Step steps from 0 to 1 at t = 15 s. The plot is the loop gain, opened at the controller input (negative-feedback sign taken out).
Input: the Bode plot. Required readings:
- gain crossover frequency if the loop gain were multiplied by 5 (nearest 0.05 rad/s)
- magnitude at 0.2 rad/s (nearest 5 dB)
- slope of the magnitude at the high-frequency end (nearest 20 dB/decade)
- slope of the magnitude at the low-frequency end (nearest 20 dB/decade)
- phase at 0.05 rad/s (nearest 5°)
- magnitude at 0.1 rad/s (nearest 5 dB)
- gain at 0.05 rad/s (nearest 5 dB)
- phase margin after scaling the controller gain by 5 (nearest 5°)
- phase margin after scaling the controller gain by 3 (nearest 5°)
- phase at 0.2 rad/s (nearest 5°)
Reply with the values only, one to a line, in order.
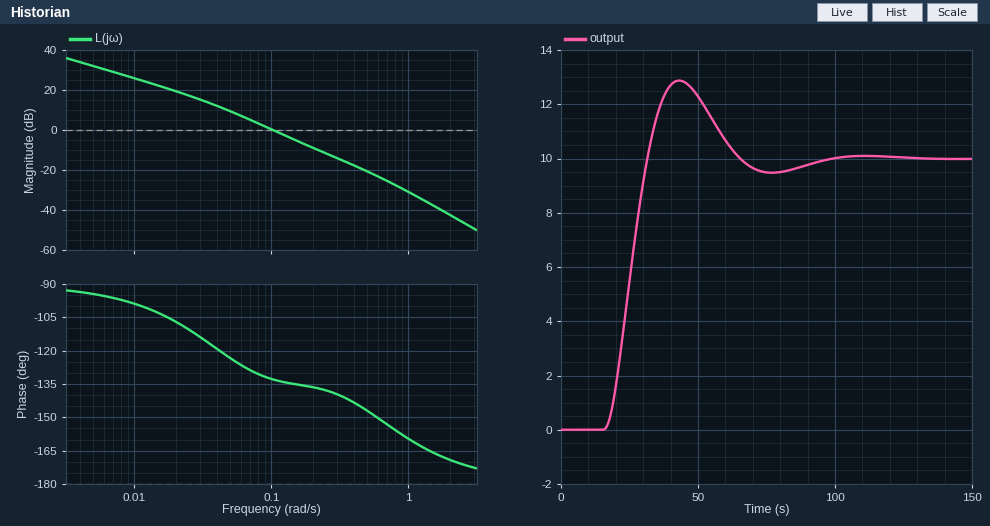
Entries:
0.30 rad/s
-10 dB
-40 dB/decade
-20 dB/decade
-125°
0 dB
10 dB
40°
45°
-135°
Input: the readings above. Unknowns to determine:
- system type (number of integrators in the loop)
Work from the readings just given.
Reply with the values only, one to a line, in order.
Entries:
1
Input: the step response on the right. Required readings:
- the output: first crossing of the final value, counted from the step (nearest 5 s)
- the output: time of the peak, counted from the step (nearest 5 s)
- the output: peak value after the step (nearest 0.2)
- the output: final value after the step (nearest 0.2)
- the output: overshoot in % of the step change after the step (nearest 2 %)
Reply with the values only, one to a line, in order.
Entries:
15 s
30 s
12.8
10.0
28 %
